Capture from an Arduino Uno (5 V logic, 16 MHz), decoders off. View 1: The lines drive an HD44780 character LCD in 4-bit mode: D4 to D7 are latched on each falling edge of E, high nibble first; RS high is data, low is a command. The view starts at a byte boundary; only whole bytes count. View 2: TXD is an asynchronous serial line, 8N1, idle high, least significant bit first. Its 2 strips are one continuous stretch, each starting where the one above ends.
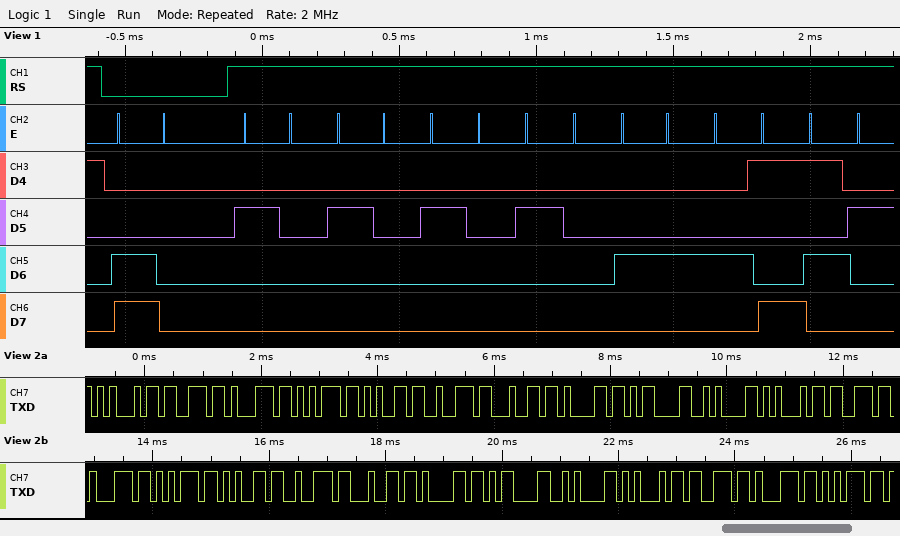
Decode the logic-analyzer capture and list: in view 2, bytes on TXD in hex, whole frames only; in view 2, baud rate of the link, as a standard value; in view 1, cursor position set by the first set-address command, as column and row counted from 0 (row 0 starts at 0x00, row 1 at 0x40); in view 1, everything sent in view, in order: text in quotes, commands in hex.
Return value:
45 73 71 75 65 72 64 61 0D 0A 45 73 71 75 65 72 64 61 0D 0A 45 73 71 75
9600 baud
column 0, row 1
0xC0 "    DIR"
